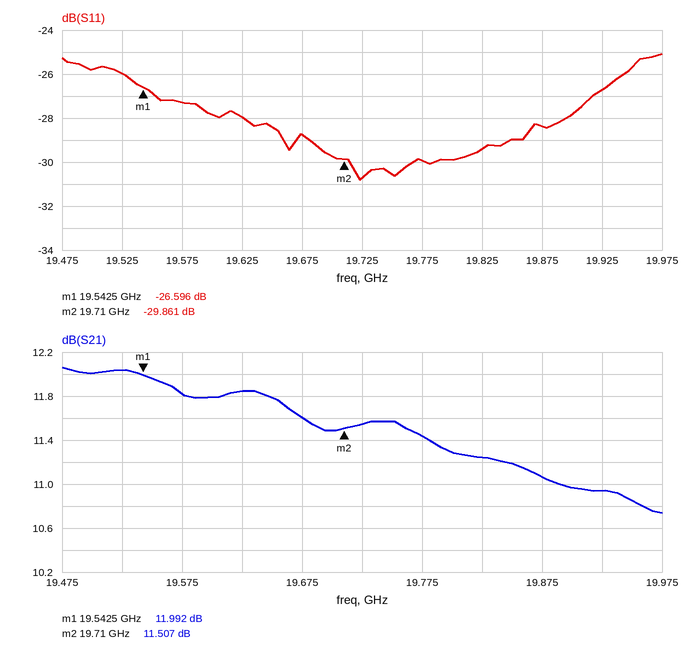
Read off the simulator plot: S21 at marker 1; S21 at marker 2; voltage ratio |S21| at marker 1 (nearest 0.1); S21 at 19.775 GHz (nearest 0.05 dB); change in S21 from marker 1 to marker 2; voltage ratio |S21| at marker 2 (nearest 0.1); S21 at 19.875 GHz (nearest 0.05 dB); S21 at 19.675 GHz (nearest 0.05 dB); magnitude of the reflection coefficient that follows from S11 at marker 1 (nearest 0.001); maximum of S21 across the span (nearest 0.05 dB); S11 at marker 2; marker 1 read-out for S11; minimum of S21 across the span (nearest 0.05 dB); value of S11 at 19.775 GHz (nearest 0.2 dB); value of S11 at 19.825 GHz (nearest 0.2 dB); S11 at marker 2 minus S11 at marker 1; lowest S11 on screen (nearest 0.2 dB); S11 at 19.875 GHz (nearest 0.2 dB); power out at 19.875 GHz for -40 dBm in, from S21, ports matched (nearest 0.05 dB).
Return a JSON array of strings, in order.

["11.992 dB", "11.507 dB", "4.0", "11.45 dB", "-0.485 dB", "3.8", "11.05 dB", "11.60 dB", "0.047", "12.05 dB", "-29.861 dB", "-26.596 dB", "10.75 dB", "-30.0 dB", "-29.4 dB", "-3.265 dB", "-30.8 dB", "-28.4 dB", "-28.95 dBm"]
